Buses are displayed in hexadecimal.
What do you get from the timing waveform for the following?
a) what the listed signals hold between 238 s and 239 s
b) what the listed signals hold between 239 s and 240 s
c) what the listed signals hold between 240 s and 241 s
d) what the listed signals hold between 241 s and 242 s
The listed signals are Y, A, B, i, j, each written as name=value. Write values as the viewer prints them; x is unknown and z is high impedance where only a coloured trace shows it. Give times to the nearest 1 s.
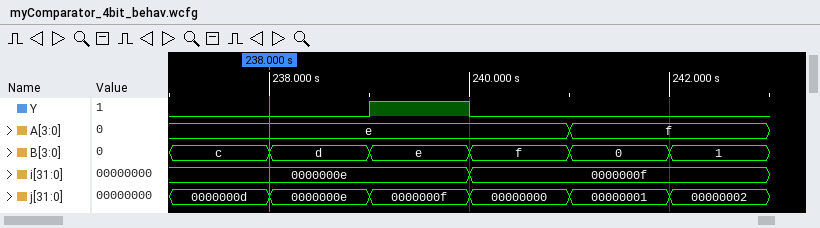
Y=0, A=e, B=d, i=0000000e, j=0000000e
Y=1, A=e, B=e, i=0000000e, j=0000000f
Y=0, A=e, B=f, i=0000000f, j=00000000
Y=0, A=f, B=0, i=0000000f, j=00000001
